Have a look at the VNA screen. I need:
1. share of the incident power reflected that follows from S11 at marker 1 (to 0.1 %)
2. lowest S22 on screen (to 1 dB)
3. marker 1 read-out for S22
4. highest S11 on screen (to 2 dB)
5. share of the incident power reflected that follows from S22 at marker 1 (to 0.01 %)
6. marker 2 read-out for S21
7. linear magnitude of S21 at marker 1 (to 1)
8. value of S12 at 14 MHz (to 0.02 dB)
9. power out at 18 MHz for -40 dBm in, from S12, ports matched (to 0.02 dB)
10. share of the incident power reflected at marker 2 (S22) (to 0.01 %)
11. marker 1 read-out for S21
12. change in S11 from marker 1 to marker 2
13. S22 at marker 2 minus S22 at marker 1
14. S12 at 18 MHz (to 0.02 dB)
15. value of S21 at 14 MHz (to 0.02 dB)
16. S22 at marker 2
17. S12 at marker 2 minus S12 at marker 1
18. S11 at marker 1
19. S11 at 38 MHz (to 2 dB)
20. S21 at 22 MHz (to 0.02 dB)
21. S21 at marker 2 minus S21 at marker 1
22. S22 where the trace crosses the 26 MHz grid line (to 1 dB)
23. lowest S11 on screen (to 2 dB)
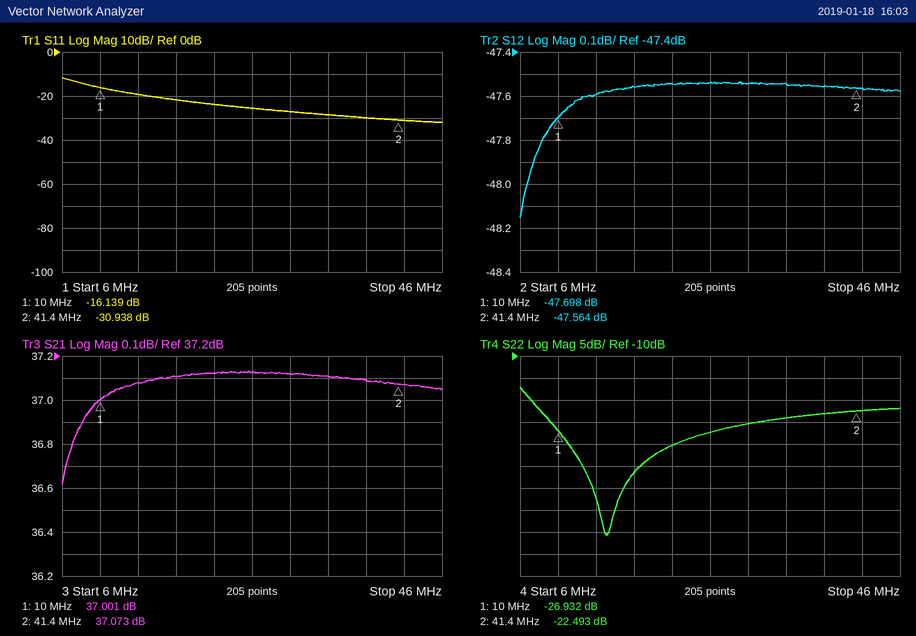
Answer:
2.4 %
-51 dB
-26.932 dB
-12 dB
0.20 %
37.073 dB
71
-47.60 dB
-87.56 dBm
0.56 %
37.001 dB
-14.799 dB
4.439 dB
-47.56 dB
37.08 dB
-22.493 dB
0.134 dB
-16.139 dB
-30 dB
37.12 dB
0.072 dB
-27 dB
-32 dB
